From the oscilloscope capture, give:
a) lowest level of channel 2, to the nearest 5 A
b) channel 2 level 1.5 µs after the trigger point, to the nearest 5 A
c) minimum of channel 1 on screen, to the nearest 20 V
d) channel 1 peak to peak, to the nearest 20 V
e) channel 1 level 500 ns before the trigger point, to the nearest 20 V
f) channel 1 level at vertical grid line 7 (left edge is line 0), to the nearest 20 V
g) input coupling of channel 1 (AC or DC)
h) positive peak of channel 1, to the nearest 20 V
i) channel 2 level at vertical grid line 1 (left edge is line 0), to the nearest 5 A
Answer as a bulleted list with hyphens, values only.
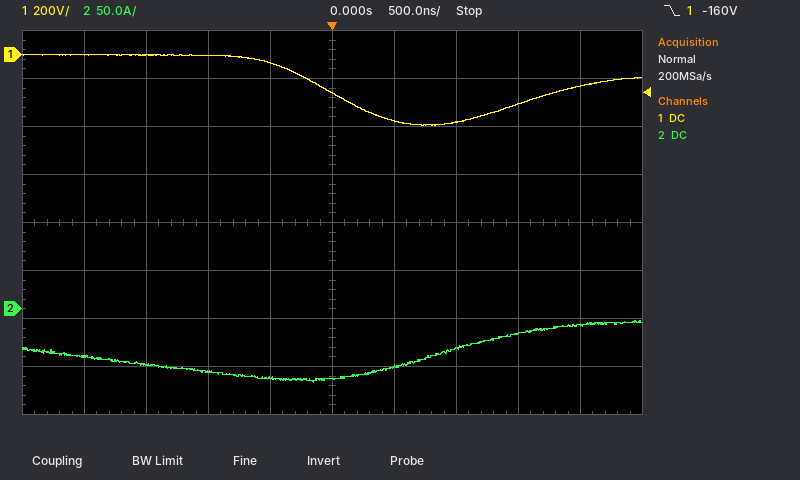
- -75 A
- -25 A
- -300 V
- 300 V
- -40 V
- -280 V
- DC
- 0 V
- -50 A
